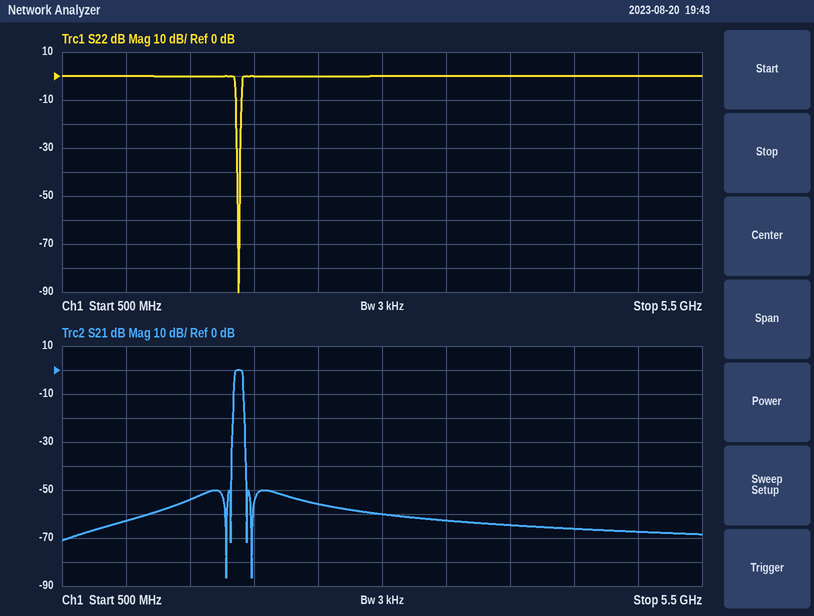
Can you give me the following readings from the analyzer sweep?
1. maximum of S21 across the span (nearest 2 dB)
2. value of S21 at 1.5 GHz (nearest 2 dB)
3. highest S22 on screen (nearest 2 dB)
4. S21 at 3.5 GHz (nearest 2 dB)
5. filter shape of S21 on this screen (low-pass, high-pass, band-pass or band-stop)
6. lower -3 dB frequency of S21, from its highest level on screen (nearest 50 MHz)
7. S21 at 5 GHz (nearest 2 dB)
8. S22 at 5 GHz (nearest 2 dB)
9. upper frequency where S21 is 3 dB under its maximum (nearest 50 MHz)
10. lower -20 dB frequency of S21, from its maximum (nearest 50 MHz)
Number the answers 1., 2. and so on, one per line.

1. 0 dB
2. -54 dB
3. 0 dB
4. -62 dB
5. band-pass
6. 1.85 GHz
7. -68 dB
8. 0 dB
9. 1.90 GHz
10. 1.85 GHz
